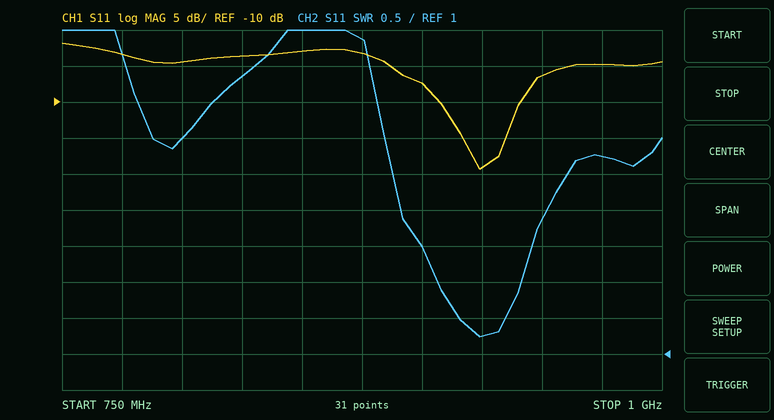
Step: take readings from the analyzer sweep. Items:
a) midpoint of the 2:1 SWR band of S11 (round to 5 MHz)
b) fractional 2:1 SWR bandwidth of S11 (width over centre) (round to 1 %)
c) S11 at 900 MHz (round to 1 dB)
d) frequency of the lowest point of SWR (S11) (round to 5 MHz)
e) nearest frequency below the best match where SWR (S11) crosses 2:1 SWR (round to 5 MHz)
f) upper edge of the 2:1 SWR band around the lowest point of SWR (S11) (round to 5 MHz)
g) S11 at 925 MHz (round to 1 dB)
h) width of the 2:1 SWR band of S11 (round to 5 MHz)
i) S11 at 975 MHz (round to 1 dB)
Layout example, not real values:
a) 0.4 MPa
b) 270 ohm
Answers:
a) 925 MHz
b) 4 %
c) -7 dB
d) 925 MHz
e) 905 MHz
f) 940 MHz
g) -19 dB
h) 35 MHz
i) -5 dB
